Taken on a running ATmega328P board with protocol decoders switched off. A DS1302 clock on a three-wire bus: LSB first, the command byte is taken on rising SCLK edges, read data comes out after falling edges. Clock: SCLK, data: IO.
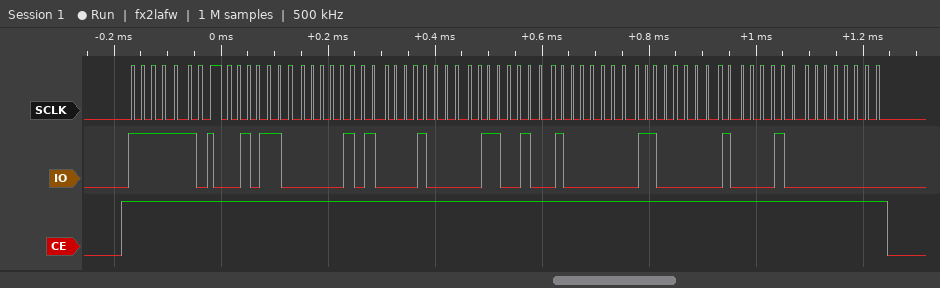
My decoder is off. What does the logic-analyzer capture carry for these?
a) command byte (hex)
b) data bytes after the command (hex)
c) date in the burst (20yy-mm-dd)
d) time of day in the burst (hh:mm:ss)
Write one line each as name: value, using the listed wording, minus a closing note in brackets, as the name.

command byte: 0xBF
data bytes after the command: 34 50 08 26 01 03 21 00
date in the burst: 2021-01-26
time of day in the burst: 08:50:34
